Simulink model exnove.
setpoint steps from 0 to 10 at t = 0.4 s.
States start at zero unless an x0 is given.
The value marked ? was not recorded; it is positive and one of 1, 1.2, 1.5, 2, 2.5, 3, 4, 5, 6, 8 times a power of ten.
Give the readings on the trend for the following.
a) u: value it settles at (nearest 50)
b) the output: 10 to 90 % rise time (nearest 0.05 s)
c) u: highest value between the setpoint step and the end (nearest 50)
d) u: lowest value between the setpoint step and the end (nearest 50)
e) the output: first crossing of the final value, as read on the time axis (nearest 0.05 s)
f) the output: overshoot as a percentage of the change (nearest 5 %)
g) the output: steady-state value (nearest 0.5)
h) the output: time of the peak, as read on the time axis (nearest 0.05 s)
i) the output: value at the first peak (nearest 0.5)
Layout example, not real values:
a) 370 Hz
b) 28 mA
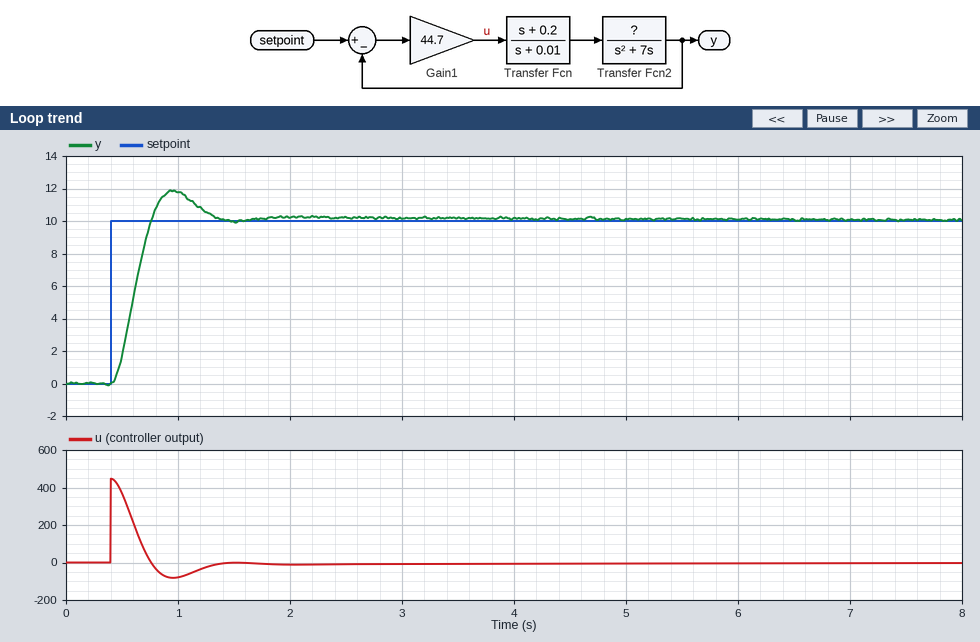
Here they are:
a) 0
b) 0.25 s
c) 450
d) -100
e) 0.75 s
f) 20 %
g) 10.0
h) 0.95 s
i) 12.0
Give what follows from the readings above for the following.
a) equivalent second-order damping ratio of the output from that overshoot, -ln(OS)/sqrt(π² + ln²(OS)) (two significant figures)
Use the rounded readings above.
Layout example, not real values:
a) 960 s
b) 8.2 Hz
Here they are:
a) 0.46
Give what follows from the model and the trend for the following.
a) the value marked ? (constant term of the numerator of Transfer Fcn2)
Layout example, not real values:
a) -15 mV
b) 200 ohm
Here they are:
a) 1
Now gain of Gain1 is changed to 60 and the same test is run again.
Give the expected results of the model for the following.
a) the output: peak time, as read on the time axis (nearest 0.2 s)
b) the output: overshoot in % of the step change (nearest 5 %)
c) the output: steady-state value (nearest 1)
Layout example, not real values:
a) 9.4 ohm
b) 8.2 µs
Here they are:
a) 0.8 s
b) 25 %
c) 10
